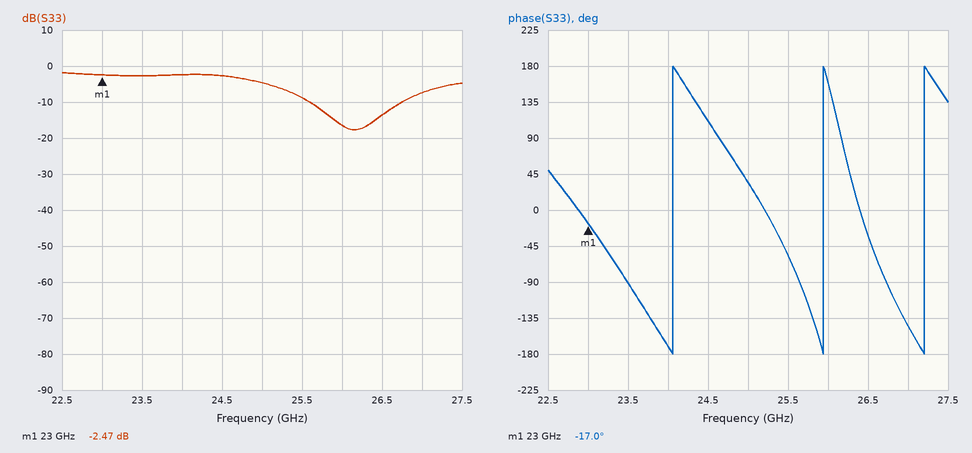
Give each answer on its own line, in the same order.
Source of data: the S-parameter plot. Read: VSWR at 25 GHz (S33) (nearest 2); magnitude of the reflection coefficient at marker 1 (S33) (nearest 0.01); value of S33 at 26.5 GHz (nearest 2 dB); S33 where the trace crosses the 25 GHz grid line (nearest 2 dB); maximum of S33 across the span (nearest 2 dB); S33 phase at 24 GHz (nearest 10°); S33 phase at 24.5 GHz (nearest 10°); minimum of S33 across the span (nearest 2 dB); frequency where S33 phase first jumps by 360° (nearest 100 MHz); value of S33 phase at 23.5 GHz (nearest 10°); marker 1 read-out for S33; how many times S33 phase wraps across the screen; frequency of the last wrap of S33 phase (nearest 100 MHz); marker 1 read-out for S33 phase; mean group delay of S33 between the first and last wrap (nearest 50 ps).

4
0.75
-14 dB
-4 dB
-2 dB
-170°
110°
-18 dB
24.1 GHz
-90°
-2.47 dB
3
27.2 GHz
-17.0°
650 ps
